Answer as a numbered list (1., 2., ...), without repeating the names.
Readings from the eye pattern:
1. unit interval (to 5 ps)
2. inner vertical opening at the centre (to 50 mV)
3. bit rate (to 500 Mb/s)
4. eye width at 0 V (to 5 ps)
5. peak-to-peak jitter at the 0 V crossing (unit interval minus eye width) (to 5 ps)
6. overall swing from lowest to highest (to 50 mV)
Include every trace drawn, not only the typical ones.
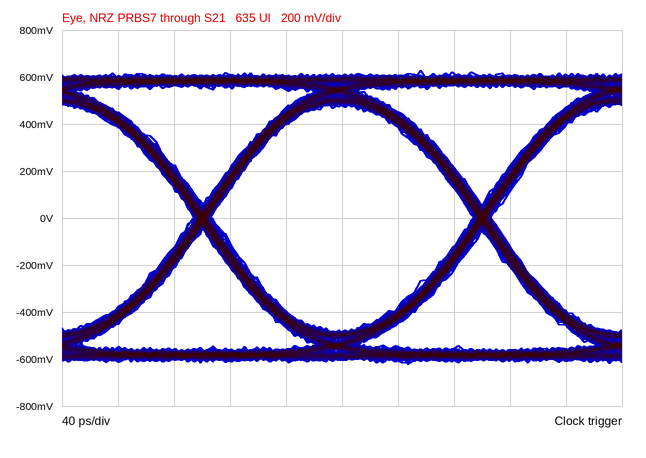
1. 200 ps
2. 950 mV
3. 5.0 Gb/s
4. 185 ps
5. 15 ps
6. 1.25 V
